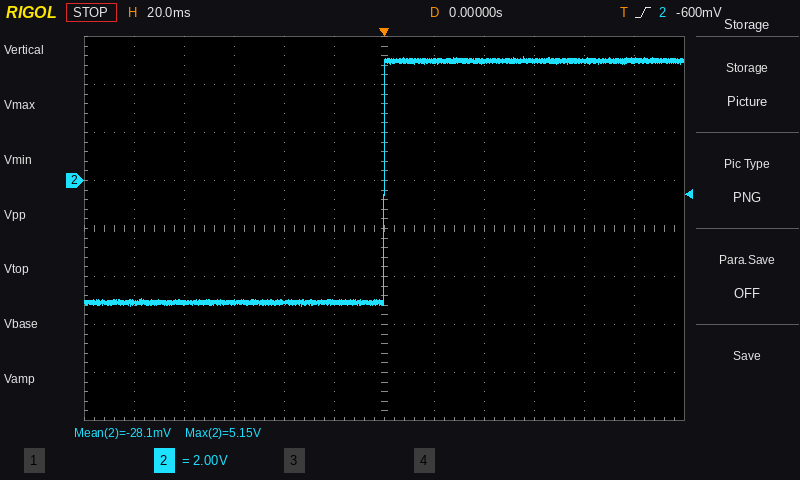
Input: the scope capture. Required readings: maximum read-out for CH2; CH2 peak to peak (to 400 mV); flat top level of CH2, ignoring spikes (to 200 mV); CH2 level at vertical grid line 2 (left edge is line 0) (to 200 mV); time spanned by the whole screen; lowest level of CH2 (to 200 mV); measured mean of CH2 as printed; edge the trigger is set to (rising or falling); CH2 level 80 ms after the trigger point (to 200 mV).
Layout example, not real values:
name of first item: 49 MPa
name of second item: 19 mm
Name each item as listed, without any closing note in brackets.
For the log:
maximum read-out for CH2: 5.15 V
CH2 peak to peak: 10.4 V
flat top level of CH2, ignoring spikes: 5.0 V
CH2 level at vertical grid line 2 (left edge is line 0): -5.0 V
time spanned by the whole screen: 240 ms
lowest level of CH2: -5.2 V
measured mean of CH2 as printed: -28.1 mV
edge the trigger is set to: rising
CH2 level 80 ms after the trigger point: 5.0 V
